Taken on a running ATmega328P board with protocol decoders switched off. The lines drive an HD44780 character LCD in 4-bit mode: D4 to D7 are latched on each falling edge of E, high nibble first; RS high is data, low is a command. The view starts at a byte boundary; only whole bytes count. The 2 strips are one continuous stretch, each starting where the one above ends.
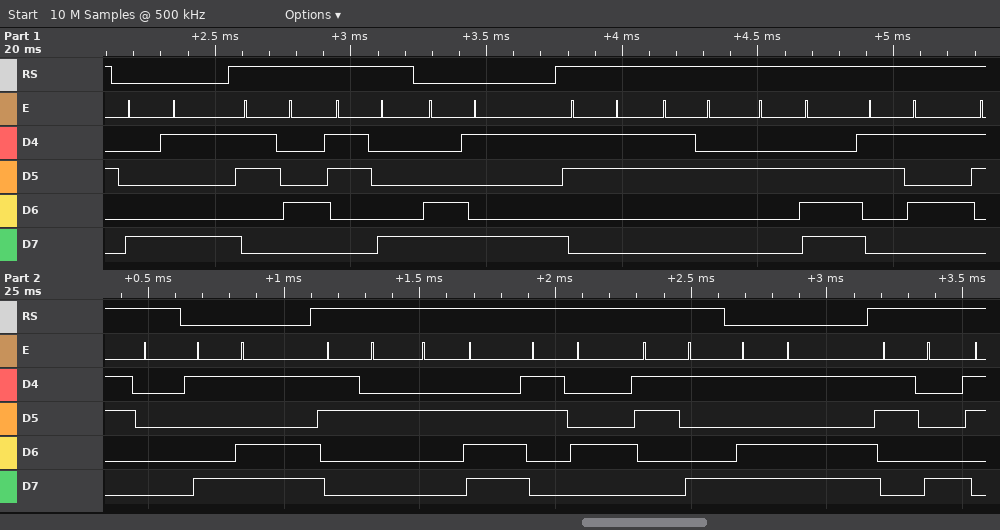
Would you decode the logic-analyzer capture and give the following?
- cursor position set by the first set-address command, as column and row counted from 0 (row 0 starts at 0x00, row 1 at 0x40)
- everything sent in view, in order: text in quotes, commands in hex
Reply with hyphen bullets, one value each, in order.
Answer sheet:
- column 9, row 0
- 0x89 "48" 0xC9 "32.50" 0x9D "2.49" 0xDD "8"
